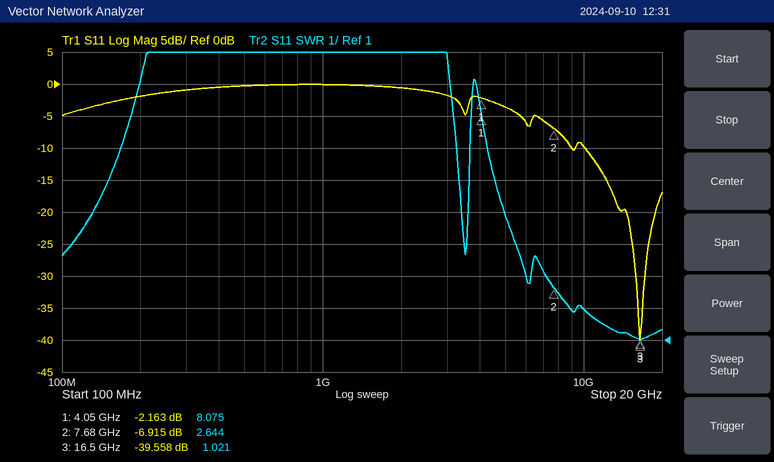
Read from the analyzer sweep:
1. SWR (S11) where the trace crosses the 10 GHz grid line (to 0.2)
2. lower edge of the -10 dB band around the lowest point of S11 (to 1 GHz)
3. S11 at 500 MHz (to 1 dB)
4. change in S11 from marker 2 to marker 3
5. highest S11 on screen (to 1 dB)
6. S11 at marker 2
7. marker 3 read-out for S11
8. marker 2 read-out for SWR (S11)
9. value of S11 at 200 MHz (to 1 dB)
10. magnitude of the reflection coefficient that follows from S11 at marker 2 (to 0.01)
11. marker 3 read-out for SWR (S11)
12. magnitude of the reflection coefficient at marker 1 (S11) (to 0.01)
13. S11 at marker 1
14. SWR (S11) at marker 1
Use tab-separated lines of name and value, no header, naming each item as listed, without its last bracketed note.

SWR (S11) where the trace crosses the 10 GHz grid line	2.0
lower edge of the -10 dB band around the lowest point of S11	10 GHz
S11 at 500 MHz	0 dB
change in S11 from marker 2 to marker 3	-32.643 dB
highest S11 on screen	0 dB
S11 at marker 2	-6.915 dB
marker 3 read-out for S11	-39.558 dB
marker 2 read-out for SWR	2.644
value of S11 at 200 MHz	-2 dB
magnitude of the reflection coefficient that follows from S11 at marker 2	0.45
marker 3 read-out for SWR	1.021
magnitude of the reflection coefficient at marker 1 (S11)	0.78
S11 at marker 1	-2.163 dB
SWR (S11) at marker 1	8.075
